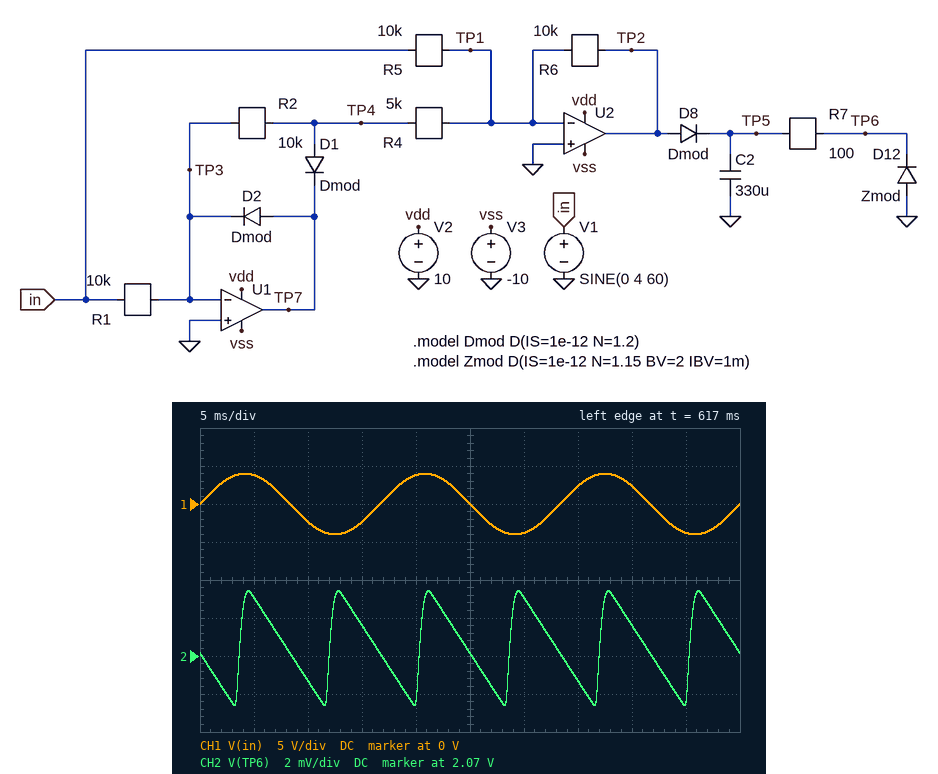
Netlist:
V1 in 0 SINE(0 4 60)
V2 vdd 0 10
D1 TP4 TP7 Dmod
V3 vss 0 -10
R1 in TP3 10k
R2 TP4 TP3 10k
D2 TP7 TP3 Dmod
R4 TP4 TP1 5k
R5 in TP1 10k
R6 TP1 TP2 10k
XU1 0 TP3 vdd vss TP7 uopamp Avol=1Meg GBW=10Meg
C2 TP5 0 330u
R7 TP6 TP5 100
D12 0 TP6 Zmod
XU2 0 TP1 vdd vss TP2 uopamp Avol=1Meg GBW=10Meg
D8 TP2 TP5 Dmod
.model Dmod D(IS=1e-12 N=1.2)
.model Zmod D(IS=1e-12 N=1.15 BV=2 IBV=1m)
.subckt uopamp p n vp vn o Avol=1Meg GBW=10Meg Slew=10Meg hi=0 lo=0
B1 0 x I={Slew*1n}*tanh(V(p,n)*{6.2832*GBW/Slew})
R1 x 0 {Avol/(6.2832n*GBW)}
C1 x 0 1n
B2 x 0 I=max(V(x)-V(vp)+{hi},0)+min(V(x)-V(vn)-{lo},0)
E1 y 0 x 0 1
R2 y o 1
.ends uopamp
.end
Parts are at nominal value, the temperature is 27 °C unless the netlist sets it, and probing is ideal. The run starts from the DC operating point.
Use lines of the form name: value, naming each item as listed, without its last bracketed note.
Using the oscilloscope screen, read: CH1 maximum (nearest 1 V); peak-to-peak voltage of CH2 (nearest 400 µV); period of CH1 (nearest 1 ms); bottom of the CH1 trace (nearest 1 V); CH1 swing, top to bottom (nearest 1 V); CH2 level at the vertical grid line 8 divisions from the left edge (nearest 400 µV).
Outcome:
CH1 maximum: 4 V
peak-to-peak voltage of CH2: 6.0 mV
period of CH1: 17 ms
bottom of the CH1 trace: -4 V
CH1 swing, top to bottom: 8 V
CH2 level at the vertical grid line 8 divisions from the left edge: 2.0716 V
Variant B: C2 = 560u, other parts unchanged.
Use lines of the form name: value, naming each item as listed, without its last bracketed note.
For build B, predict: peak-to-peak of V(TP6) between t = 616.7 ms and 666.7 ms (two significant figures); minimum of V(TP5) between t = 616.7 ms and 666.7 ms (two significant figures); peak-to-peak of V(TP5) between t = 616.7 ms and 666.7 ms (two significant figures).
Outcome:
peak-to-peak of V(TP6) between t = 616.7 ms and 666.7 ms: 3.6 mV
minimum of V(TP5) between t = 616.7 ms and 666.7 ms: 3.1 V
peak-to-peak of V(TP5) between t = 616.7 ms and 666.7 ms: 140 mV
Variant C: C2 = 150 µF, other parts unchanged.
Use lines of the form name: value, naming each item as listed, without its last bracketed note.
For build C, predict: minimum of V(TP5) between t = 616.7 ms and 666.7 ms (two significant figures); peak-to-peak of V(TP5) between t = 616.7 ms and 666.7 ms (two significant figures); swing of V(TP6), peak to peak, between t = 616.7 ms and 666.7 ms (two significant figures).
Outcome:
minimum of V(TP5) between t = 616.7 ms and 666.7 ms: 2.8 V
peak-to-peak of V(TP5) between t = 616.7 ms and 666.7 ms: 430 mV
swing of V(TP6), peak to peak, between t = 616.7 ms and 666.7 ms: 13 mV
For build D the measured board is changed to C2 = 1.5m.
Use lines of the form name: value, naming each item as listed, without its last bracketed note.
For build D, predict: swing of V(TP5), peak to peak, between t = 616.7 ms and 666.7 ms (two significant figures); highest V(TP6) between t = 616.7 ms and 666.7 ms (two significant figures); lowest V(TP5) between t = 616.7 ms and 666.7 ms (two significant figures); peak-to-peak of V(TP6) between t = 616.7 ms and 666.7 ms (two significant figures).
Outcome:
swing of V(TP5), peak to peak, between t = 616.7 ms and 666.7 ms: 53 mV
highest V(TP6) between t = 616.7 ms and 666.7 ms: 2.1 V
lowest V(TP5) between t = 616.7 ms and 666.7 ms: 3.2 V
peak-to-peak of V(TP6) between t = 616.7 ms and 666.7 ms: 1.4 mV
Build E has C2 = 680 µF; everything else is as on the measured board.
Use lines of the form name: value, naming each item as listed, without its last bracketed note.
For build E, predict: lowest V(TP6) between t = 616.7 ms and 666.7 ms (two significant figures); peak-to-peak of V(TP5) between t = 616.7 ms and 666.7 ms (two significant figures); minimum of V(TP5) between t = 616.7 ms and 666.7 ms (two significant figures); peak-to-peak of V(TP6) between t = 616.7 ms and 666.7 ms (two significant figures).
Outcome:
lowest V(TP6) between t = 616.7 ms and 666.7 ms: 2.1 V
peak-to-peak of V(TP5) between t = 616.7 ms and 666.7 ms: 110 mV
minimum of V(TP5) between t = 616.7 ms and 666.7 ms: 3.1 V
peak-to-peak of V(TP6) between t = 616.7 ms and 666.7 ms: 3.0 mV
